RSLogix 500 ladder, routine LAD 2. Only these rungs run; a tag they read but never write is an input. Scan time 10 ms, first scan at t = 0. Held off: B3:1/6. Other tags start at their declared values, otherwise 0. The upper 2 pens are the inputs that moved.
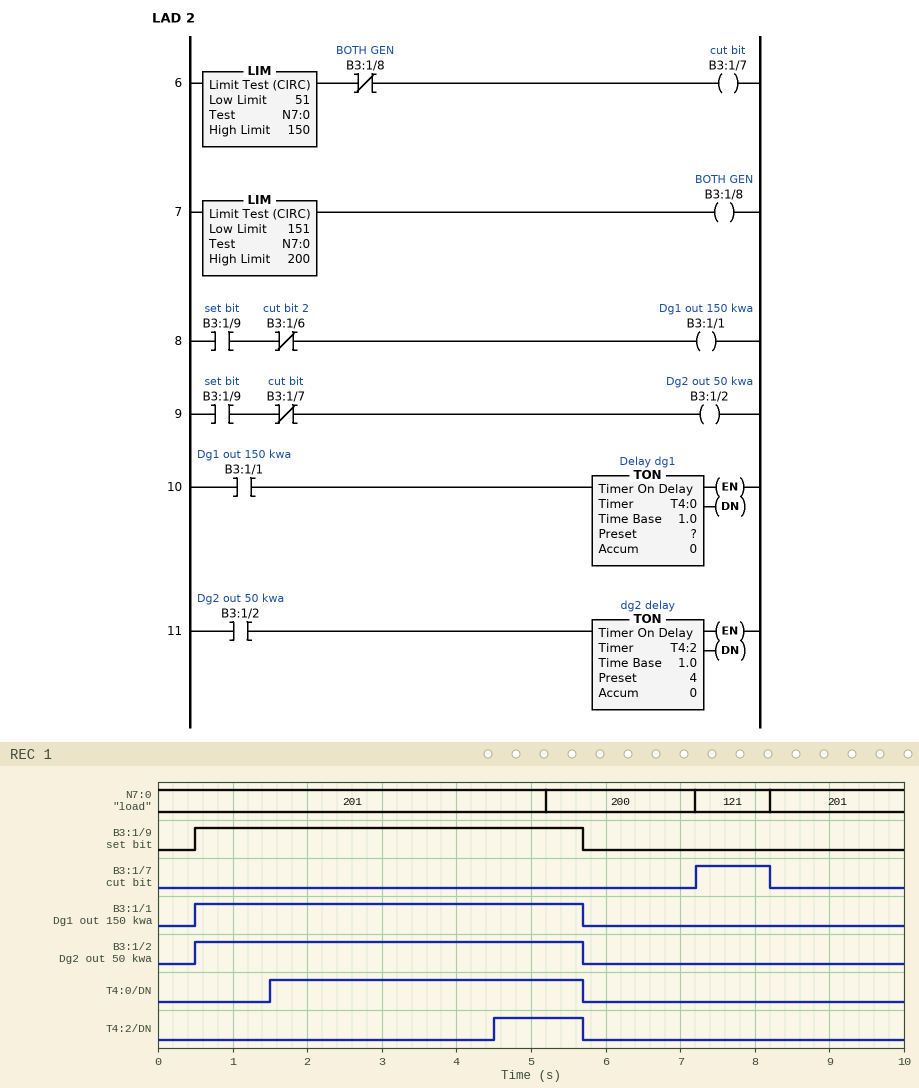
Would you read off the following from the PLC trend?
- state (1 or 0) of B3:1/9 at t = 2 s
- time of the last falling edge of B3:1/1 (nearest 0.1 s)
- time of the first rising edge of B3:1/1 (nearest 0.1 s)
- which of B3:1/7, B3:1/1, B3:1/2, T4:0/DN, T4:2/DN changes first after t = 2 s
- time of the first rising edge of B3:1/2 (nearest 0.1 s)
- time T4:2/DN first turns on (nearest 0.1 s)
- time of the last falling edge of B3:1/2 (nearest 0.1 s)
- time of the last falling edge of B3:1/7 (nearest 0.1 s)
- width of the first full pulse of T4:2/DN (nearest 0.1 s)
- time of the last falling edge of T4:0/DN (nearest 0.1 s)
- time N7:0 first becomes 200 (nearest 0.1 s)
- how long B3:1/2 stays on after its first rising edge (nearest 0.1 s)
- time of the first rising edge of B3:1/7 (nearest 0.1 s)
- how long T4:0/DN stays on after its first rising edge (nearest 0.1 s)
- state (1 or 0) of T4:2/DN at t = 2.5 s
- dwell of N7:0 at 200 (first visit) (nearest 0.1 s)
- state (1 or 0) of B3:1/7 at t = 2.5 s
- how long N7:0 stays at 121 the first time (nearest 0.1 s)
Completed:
1
5.7 s
0.5 s
T4:2/DN
0.5 s
4.5 s
5.7 s
8.2 s
1.2 s
5.7 s
5.2 s
5.2 s
7.2 s
4.2 s
0
2.0 s
0
1.0 s
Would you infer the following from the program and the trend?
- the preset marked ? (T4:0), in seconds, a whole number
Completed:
1 s
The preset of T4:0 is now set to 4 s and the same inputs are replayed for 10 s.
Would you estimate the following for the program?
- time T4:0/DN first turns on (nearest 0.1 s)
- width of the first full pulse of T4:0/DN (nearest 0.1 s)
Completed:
4.5 s
1.2 s
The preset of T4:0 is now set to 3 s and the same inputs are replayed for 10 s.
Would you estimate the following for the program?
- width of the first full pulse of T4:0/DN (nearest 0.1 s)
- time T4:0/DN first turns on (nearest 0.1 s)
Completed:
2.2 s
3.5 s
